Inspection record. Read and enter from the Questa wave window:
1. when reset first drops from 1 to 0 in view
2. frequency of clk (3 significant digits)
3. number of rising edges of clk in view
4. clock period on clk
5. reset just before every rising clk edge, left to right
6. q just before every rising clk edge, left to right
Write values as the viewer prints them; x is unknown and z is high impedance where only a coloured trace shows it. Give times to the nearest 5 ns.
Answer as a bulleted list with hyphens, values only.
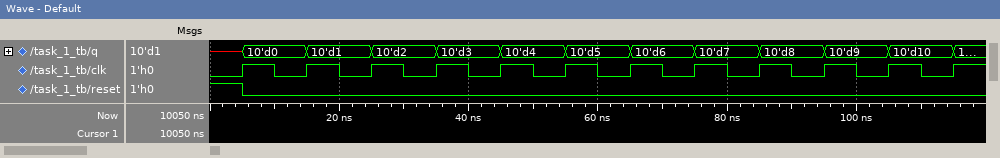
- 5 ns
- 100 MHz
- 12
- 10 ns
- 1 0 0 0 0 0 0 0 0 0 0 0
- x, 10'd0, 10'd1, 10'd2, 10'd3, 10'd4, 10'd5, 10'd6, 10'd7, 10'd8, 10'd9, 10'd10
